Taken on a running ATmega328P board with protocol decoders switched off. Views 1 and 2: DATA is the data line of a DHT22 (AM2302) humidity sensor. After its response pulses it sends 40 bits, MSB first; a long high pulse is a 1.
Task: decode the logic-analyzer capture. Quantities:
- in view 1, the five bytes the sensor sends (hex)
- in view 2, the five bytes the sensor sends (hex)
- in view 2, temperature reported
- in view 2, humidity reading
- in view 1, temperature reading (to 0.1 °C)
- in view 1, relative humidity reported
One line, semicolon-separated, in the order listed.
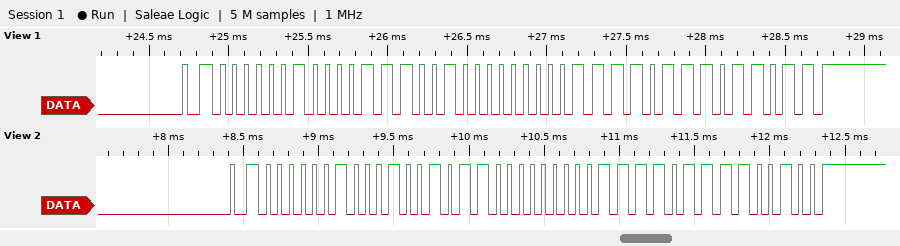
02 1C 80 3D DB; 02 25 80 3D E4; -6.1 °C; 54.9 %; -6.1 °C; 54.0 %
